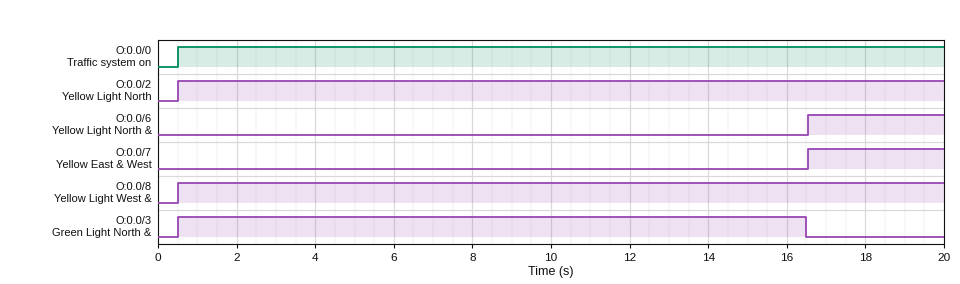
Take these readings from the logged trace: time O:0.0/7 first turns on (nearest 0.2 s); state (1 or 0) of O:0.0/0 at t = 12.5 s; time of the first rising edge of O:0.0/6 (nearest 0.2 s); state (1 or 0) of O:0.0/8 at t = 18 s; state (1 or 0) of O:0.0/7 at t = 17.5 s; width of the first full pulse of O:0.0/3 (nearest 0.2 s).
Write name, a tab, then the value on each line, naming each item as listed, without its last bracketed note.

time O:0.0/7 first turns on	16.6 s
state (1 or 0) of O:0.0/0 at t = 12.5 s	1
time of the first rising edge of O:0.0/6	16.6 s
state (1 or 0) of O:0.0/8 at t = 18 s	1
state (1 or 0) of O:0.0/7 at t = 17.5 s	1
width of the first full pulse of O:0.0/3	16.0 s
